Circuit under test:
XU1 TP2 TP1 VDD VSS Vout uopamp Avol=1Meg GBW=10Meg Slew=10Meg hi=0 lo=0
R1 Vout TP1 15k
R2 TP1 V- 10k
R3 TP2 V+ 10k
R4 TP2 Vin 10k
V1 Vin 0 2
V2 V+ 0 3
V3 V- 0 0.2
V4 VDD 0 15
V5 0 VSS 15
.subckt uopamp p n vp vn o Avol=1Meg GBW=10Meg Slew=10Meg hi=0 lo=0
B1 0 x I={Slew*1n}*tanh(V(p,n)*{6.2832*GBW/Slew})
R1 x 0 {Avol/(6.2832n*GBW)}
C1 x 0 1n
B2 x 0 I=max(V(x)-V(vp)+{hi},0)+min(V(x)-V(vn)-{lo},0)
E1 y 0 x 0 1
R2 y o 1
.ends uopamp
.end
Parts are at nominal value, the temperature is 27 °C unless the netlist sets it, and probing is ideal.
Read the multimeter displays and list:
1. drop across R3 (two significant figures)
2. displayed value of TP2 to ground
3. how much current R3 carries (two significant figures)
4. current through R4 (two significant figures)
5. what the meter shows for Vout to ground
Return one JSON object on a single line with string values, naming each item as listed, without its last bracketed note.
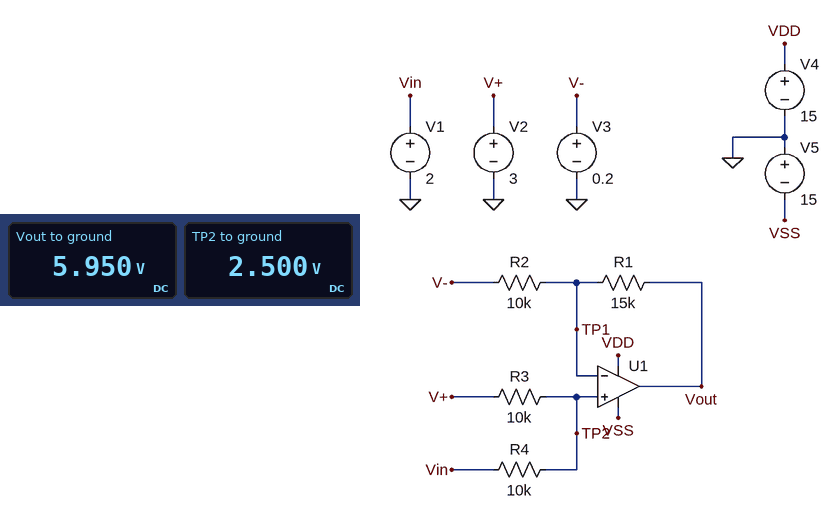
{"drop across R3": "500 mV", "displayed value of TP2 to ground": "2.500 V", "how much current R3 carries": "50 µA", "current through R4": "50 µA", "what the meter shows for Vout to ground": "5.950 V"}
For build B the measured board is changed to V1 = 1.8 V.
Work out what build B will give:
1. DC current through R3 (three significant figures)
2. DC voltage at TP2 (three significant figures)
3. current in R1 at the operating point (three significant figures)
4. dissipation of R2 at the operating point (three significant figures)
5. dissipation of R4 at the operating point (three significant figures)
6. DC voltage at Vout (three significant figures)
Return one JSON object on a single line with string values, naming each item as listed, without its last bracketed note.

{"DC current through R3": "60.0 µA", "DC voltage at TP2": "2.40 V", "current in R1 at the operating point": "220 µA", "dissipation of R2 at the operating point": "484 µW", "dissipation of R4 at the operating point": "36.0 µW", "DC voltage at Vout": "5.70 V"}
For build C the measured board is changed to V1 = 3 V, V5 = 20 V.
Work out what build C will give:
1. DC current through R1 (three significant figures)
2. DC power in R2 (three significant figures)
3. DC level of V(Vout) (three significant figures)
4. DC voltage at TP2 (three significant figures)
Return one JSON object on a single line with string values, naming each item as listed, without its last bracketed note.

{"DC current through R1": "280 µA", "DC power in R2": "784 µW", "DC level of V(Vout)": "7.20 V", "DC voltage at TP2": "3.00 V"}
